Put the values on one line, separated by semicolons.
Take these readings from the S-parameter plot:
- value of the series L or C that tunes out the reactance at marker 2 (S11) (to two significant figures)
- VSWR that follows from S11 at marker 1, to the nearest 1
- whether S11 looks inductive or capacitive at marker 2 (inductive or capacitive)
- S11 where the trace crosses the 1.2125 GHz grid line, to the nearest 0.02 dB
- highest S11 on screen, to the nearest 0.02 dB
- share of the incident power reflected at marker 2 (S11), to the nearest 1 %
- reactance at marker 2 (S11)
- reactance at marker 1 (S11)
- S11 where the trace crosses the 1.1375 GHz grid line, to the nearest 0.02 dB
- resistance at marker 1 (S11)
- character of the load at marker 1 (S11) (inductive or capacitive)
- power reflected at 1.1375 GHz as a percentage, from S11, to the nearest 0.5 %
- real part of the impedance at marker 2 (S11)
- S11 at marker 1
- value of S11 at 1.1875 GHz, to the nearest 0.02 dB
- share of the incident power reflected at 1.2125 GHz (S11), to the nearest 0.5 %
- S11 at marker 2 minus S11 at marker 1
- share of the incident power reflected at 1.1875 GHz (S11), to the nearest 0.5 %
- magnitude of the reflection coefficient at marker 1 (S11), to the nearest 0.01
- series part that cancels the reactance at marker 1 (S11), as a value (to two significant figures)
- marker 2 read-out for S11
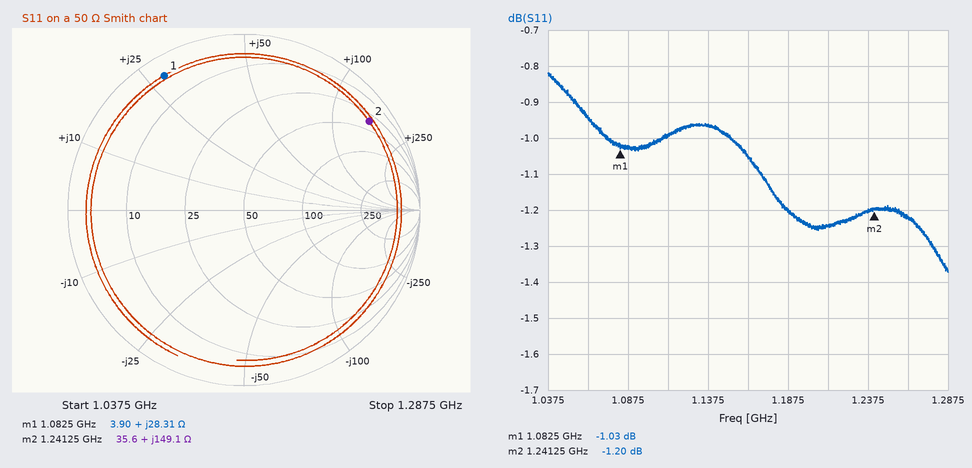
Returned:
860 fF; 17; inductive; -1.24 dB; -0.82 dB; 76 %; +149.1 Ω; +28.31 Ω; -0.96 dB; 3.90 Ω; inductive; 80.0 %; 35.6 Ω; -1.03 dB; -1.20 dB; 75.0 %; -0.17 dB; 76.0 %; 0.89; 5.2 pF; -1.20 dB
